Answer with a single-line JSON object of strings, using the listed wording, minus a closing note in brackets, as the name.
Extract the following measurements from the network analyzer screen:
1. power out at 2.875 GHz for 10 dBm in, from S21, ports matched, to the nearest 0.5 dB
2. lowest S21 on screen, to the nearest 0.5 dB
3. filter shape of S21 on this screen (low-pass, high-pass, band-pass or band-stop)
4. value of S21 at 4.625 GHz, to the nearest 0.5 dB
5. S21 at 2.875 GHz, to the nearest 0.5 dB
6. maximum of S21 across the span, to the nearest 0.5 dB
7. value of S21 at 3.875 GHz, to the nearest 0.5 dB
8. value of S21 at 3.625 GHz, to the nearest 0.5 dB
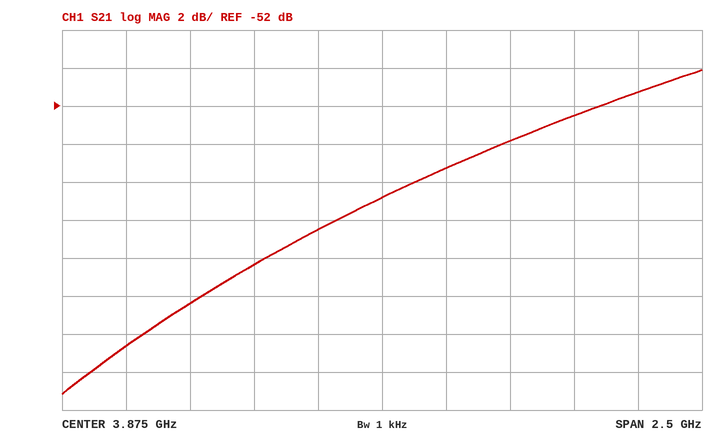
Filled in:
{"power out at 2.875 GHz for 10 dBm in, from S21, ports matched, to the nearest 0.5 dB": "-54.5 dBm", "lowest S21 on screen, to the nearest 0.5 dB": "-67.0 dB", "filter shape of S21 on this screen": "high-pass", "value of S21 at 4.625 GHz, to the nearest 0.5 dB": "-52.5 dB", "S21 at 2.875 GHz, to the nearest 0.5 dB": "-64.5 dB", "maximum of S21 across the span, to the nearest 0.5 dB": "-50.0 dB", "value of S21 at 3.875 GHz, to the nearest 0.5 dB": "-57.0 dB", "value of S21 at 3.625 GHz, to the nearest 0.5 dB": "-58.5 dB"}
